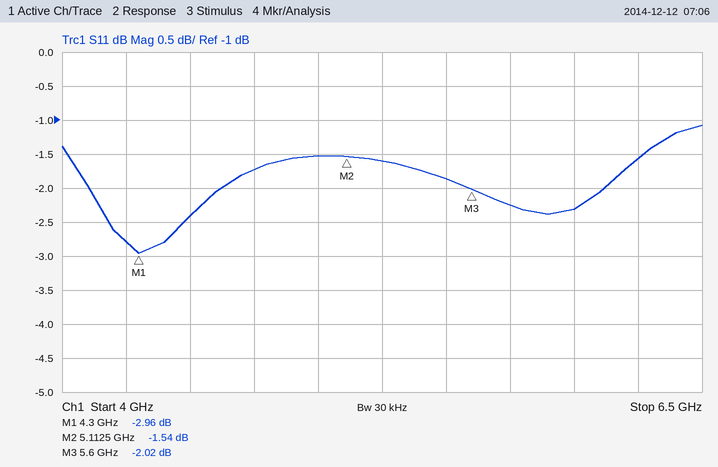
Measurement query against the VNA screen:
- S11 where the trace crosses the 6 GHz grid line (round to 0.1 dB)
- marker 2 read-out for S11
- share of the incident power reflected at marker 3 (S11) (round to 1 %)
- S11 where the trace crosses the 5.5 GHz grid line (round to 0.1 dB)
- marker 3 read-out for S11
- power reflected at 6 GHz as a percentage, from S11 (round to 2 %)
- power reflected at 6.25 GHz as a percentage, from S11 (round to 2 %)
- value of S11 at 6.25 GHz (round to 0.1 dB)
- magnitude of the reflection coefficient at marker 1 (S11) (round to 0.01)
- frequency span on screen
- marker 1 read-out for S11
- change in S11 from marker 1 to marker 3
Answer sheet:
-2.3 dB
-1.54 dB
63 %
-1.9 dB
-2.02 dB
58 %
70 %
-1.6 dB
0.71
2.5 GHz
-2.96 dB
0.94 dB
